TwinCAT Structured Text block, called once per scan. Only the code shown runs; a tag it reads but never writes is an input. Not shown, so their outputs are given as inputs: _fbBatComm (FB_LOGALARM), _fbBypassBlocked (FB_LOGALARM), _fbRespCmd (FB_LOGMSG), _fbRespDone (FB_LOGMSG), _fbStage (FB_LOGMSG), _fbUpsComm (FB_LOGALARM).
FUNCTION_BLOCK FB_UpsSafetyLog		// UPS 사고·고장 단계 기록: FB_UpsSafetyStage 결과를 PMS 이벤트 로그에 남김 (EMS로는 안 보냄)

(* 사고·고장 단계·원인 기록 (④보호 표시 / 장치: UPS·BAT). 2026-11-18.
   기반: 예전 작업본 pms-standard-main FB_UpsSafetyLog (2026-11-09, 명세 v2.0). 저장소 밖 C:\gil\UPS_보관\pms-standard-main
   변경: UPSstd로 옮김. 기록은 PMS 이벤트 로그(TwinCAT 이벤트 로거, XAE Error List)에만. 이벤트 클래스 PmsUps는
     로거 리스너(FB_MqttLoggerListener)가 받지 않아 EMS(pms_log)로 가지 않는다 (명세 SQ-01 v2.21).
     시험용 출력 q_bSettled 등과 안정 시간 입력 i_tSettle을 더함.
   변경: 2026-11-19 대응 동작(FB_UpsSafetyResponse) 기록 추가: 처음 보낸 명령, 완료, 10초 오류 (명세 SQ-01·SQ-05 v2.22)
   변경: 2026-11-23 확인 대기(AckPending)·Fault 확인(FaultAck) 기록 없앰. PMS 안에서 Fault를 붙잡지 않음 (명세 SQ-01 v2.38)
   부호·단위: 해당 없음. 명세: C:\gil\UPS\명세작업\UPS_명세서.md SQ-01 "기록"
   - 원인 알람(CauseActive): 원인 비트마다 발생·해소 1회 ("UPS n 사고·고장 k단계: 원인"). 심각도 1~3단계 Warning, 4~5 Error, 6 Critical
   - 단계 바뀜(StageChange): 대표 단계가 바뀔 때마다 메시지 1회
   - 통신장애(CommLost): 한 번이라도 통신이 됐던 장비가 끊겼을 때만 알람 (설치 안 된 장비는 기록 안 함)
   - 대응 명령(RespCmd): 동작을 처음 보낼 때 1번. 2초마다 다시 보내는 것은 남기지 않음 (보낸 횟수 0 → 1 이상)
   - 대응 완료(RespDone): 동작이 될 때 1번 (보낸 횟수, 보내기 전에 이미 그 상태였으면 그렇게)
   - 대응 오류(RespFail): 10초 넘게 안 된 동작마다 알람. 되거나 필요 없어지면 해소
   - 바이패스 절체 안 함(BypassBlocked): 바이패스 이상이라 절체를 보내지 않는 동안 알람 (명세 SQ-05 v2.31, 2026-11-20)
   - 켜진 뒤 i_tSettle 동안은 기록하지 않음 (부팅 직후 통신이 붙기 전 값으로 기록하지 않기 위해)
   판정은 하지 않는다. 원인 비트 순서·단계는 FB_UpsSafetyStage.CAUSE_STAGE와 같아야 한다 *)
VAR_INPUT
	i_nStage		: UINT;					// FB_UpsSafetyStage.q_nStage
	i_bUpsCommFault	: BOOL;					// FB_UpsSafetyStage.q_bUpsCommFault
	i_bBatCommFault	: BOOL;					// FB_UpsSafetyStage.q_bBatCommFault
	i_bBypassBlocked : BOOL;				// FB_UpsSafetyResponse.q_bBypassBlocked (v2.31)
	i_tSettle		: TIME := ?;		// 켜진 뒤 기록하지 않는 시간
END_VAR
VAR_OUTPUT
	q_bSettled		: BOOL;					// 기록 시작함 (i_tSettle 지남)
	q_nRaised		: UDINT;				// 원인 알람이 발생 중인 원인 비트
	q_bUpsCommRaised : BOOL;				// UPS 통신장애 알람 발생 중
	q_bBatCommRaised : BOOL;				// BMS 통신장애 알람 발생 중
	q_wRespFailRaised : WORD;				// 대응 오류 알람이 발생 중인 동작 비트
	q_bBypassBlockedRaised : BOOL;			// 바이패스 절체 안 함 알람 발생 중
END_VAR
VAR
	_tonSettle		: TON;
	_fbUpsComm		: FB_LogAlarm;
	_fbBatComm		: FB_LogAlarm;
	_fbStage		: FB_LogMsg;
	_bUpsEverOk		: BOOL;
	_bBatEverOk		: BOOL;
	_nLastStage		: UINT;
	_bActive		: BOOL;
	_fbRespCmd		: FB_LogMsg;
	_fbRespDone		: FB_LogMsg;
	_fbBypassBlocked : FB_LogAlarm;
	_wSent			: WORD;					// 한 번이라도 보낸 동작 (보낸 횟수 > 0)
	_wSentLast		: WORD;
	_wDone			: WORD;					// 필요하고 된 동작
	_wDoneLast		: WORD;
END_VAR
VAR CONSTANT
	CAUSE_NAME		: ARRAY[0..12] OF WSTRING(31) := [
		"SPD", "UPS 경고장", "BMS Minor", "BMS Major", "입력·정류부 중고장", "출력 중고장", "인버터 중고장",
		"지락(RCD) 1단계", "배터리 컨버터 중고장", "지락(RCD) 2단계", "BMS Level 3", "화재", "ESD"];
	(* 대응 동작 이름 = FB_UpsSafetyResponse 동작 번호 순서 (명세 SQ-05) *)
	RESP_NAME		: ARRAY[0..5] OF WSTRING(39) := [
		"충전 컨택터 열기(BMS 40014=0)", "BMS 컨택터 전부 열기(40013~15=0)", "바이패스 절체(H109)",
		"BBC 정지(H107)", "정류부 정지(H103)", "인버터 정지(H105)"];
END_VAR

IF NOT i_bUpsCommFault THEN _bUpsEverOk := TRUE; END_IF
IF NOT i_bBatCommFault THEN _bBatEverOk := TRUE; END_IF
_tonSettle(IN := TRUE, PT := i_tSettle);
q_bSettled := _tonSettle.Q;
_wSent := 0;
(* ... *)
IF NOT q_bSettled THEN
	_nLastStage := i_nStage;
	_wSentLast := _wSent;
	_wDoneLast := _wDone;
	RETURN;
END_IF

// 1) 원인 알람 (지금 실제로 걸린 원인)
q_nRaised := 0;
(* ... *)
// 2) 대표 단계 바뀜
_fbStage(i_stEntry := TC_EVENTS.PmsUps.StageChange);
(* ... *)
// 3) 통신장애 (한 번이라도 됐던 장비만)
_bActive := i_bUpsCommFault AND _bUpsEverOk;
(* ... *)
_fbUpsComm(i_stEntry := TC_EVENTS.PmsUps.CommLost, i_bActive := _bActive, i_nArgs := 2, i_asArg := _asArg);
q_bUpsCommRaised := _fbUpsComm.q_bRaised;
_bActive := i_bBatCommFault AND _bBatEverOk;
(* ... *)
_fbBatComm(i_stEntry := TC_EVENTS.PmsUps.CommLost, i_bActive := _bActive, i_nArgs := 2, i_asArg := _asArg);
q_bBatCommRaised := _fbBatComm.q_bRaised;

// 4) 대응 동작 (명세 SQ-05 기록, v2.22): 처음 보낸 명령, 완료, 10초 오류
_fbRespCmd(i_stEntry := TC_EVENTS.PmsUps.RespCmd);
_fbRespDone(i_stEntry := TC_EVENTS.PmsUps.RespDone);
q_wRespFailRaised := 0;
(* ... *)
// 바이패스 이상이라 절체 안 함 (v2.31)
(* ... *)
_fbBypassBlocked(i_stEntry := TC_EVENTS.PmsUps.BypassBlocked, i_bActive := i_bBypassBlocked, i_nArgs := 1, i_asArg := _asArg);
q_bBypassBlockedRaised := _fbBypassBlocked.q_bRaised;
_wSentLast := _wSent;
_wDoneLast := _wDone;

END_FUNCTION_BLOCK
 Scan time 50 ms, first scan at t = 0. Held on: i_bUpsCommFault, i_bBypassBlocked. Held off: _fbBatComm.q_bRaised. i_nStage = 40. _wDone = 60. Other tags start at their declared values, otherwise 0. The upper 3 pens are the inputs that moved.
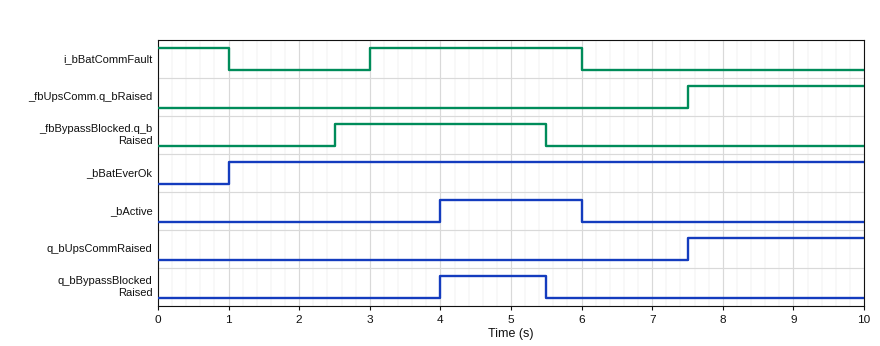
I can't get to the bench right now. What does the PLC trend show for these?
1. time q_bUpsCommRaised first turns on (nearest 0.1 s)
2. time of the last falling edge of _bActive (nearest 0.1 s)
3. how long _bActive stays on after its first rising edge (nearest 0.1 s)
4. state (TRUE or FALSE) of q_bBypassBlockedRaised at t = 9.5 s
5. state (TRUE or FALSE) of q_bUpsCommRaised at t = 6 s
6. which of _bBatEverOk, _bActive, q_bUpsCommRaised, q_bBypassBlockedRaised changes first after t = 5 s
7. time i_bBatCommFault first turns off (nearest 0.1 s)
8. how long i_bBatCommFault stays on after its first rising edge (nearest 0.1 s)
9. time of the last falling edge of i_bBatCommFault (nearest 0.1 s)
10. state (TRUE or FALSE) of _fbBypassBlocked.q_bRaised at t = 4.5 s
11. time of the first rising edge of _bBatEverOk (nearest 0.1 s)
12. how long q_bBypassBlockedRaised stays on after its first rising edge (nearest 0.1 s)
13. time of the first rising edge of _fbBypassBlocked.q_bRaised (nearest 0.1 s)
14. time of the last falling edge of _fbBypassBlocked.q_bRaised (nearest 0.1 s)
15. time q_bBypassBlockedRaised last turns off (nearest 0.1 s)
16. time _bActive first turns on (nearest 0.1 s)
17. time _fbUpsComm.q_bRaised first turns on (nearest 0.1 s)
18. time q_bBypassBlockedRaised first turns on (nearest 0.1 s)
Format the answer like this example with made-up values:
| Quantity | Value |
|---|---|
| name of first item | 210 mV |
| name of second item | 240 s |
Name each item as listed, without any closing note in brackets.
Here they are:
| Quantity | Value |
|---|---|
| time q_bUpsCommRaised first turns on | 7.5 s |
| time of the last falling edge of _bActive | 6.0 s |
| how long _bActive stays on after its first rising edge | 2.0 s |
| state (TRUE or FALSE) of q_bBypassBlockedRaised at t = 9.5 s | FALSE |
| state (TRUE or FALSE) of q_bUpsCommRaised at t = 6 s | FALSE |
| which of _bBatEverOk, _bActive, q_bUpsCommRaised, q_bBypassBlockedRaised changes first after t = 5 s | q_bBypassBlockedRaised |
| time i_bBatCommFault first turns off | 1.0 s |
| how long i_bBatCommFault stays on after its first rising edge | 3.0 s |
| time of the last falling edge of i_bBatCommFault | 6.0 s |
| state (TRUE or FALSE) of _fbBypassBlocked.q_bRaised at t = 4.5 s | TRUE |
| time of the first rising edge of _bBatEverOk | 1.0 s |
| how long q_bBypassBlockedRaised stays on after its first rising edge | 1.5 s |
| time of the first rising edge of _fbBypassBlocked.q_bRaised | 2.5 s |
| time of the last falling edge of _fbBypassBlocked.q_bRaised | 5.5 s |
| time q_bBypassBlockedRaised last turns off | 5.5 s |
| time _bActive first turns on | 4.0 s |
| time _fbUpsComm.q_bRaised first turns on | 7.5 s |
| time q_bBypassBlockedRaised first turns on | 4.0 s |
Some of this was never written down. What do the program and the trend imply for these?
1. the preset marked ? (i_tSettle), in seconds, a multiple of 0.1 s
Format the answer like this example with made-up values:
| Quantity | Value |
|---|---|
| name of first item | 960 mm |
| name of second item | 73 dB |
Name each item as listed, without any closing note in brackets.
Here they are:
| Quantity | Value |
|---|---|
| the preset marked ? (i_tSettle), in seconds, a multiple of 0.1 s | 4.0 s |
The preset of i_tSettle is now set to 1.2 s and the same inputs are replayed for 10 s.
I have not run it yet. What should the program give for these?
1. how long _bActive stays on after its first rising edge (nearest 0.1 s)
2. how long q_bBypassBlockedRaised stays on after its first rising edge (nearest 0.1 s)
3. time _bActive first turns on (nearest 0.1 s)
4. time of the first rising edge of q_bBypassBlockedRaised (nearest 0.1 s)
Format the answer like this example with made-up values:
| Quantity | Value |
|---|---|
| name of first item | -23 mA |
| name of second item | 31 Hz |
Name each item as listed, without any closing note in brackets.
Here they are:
| Quantity | Value |
|---|---|
| how long _bActive stays on after its first rising edge | 3.0 s |
| how long q_bBypassBlockedRaised stays on after its first rising edge | 3.0 s |
| time _bActive first turns on | 3.0 s |
| time of the first rising edge of q_bBypassBlockedRaised | 2.5 s |
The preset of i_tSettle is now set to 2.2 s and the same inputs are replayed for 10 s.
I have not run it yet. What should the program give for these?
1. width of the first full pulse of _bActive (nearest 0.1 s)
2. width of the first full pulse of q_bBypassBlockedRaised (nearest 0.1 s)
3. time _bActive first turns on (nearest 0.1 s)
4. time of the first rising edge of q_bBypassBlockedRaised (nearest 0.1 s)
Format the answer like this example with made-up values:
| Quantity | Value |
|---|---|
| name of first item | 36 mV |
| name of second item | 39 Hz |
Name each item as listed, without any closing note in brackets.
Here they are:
| Quantity | Value |
|---|---|
| width of the first full pulse of _bActive | 3.0 s |
| width of the first full pulse of q_bBypassBlockedRaised | 3.0 s |
| time _bActive first turns on | 3.0 s |
| time of the first rising edge of q_bBypassBlockedRaised | 2.5 s |
